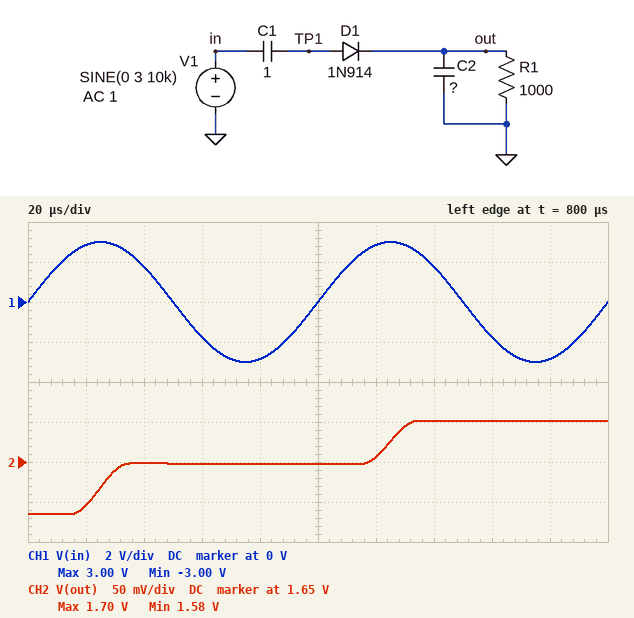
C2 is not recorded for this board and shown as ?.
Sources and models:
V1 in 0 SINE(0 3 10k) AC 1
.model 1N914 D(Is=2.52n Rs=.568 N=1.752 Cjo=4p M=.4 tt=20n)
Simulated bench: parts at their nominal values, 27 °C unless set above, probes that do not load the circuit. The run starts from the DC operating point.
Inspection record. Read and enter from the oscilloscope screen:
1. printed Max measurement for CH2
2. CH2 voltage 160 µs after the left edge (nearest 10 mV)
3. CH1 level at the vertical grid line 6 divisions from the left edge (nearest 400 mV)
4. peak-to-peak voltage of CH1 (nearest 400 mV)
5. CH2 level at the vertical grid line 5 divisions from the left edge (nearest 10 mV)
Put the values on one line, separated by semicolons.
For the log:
1.70 V; 1.70 V; 2.8 V; 6.0 V; 1.65 V
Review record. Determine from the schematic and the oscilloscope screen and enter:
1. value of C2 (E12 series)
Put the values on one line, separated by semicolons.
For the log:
180 µF
